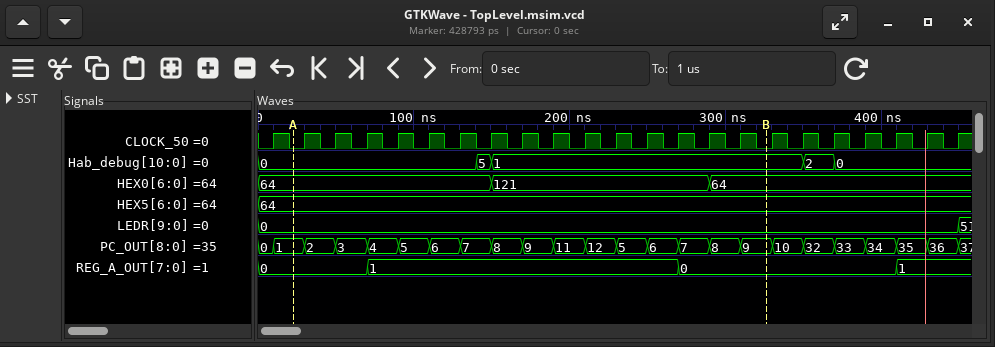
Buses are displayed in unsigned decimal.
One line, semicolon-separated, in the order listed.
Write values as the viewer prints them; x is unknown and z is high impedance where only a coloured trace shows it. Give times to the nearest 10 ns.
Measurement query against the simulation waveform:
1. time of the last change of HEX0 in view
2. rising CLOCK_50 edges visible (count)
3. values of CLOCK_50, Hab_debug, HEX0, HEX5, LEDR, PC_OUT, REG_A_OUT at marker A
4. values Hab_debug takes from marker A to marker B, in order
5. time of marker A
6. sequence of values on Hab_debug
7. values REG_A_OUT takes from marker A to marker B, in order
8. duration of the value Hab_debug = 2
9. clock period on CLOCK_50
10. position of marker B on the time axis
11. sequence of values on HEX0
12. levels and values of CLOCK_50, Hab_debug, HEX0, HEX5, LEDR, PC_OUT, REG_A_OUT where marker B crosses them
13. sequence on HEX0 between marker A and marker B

290 ns; 23; CLOCK_50=0, Hab_debug=0, HEX0=64, HEX5=64, LEDR=0, PC_OUT=1, REG_A_OUT=0; 0, 5, 1; 20 ns; 0, 5, 1, 2, 0; 0, 1, 0; 20 ns; 20 ns; 330 ns; 64, 121, 64; CLOCK_50=0, Hab_debug=1, HEX0=64, HEX5=64, LEDR=0, PC_OUT=9, REG_A_OUT=0; 64, 121, 64
